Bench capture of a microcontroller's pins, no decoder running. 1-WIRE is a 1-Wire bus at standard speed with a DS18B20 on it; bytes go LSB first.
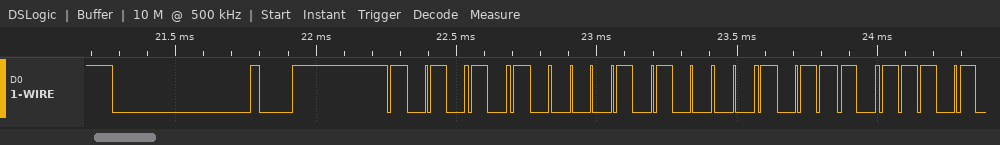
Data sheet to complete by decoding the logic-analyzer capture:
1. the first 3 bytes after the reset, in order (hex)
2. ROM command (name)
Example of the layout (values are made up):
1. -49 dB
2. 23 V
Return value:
1. 55 28 74
2. Match ROM
